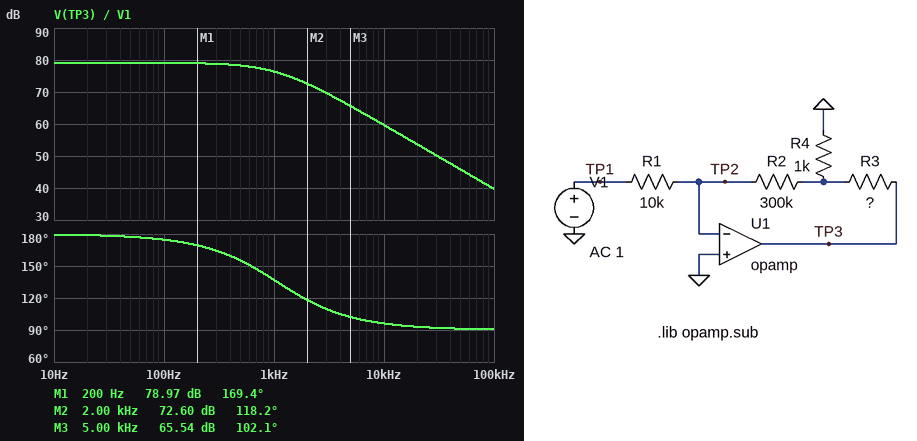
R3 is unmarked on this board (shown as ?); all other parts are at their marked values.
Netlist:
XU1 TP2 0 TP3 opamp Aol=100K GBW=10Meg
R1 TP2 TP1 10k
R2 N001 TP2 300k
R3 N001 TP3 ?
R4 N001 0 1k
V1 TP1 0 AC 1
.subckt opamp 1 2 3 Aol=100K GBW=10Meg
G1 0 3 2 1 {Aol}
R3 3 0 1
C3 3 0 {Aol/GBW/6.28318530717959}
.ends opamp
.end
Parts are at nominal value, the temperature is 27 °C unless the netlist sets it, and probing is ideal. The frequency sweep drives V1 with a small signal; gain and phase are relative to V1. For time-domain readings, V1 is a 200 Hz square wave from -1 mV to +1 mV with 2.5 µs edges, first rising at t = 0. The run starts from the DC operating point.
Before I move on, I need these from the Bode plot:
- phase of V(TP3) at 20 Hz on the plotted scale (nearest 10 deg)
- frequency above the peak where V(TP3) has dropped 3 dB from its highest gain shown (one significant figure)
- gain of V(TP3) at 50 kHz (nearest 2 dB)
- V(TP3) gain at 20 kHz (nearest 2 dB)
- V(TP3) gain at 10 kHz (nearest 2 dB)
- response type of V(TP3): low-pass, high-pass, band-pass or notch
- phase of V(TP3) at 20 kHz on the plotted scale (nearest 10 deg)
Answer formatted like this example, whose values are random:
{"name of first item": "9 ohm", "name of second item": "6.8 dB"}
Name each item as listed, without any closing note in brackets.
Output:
{"phase of V(TP3) at 20 Hz on the plotted scale": "180 deg", "frequency above the peak where V(TP3) has dropped 3 dB from its highest gain shown": "1 kHz", "gain of V(TP3) at 50 kHz": "46 dB", "V(TP3) gain at 20 kHz": "54 dB", "V(TP3) gain at 10 kHz": "60 dB", "response type of V(TP3): low-pass, high-pass, band-pass or notch": "low-pass", "phase of V(TP3) at 20 kHz on the plotted scale": "90 deg"}
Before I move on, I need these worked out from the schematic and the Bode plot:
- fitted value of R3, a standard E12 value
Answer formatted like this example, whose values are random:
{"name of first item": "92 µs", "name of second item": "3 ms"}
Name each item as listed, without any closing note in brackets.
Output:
{"fitted value of R3, a standard E12 value": "330 kΩ"}
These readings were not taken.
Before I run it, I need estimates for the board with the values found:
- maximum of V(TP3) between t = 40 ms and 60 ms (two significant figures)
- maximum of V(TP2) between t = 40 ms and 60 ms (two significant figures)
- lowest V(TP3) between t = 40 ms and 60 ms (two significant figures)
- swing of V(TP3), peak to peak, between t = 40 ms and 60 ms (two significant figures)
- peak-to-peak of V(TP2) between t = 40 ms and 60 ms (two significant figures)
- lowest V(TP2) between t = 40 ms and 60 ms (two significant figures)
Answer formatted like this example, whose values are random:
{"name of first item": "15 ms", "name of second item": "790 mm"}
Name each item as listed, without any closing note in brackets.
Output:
{"maximum of V(TP3) between t = 40 ms and 60 ms": "9.0 V", "maximum of V(TP2) between t = 40 ms and 60 ms": "1.8 mV", "lowest V(TP3) between t = 40 ms and 60 ms": "-9.0 V", "swing of V(TP3), peak to peak, between t = 40 ms and 60 ms": "18 V", "peak-to-peak of V(TP2) between t = 40 ms and 60 ms": "3.7 mV", "lowest V(TP2) between t = 40 ms and 60 ms": "-1.8 mV"}
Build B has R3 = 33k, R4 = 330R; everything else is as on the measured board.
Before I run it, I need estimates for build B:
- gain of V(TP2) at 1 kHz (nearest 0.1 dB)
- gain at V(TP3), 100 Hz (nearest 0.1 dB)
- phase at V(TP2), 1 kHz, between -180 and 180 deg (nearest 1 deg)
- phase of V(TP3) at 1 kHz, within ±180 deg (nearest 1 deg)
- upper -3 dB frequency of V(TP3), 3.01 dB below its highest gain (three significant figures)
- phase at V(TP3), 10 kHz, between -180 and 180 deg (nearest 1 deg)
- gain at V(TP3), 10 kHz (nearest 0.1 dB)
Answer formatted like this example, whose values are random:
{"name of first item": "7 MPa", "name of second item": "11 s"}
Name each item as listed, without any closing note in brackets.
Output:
{"gain of V(TP2) at 1 kHz": "-11.0 dB", "gain at V(TP3), 100 Hz": "69.4 dB", "phase at V(TP2), 1 kHz, between -180 and 180 deg": "67 deg", "phase of V(TP3) at 1 kHz, within ±180 deg": "163 deg", "upper -3 dB frequency of V(TP3), 3.01 dB below its highest gain": "3.29 kHz", "phase at V(TP3), 10 kHz, between -180 and 180 deg": "108 deg", "gain at V(TP3), 10 kHz": "59.3 dB"}
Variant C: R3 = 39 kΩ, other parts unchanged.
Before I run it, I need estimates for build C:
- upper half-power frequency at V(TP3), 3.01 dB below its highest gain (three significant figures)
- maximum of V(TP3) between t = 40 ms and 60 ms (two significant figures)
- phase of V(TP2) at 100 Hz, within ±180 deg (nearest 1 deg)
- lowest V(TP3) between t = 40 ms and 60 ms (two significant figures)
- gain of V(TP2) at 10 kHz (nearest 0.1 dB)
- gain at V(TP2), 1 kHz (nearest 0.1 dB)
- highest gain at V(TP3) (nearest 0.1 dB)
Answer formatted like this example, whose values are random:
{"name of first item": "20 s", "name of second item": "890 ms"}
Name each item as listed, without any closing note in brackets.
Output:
{"upper half-power frequency at V(TP3), 3.01 dB below its highest gain": "8.14 kHz", "maximum of V(TP3) between t = 40 ms and 60 ms": "1.2 V", "phase of V(TP2) at 100 Hz, within ±180 deg": "44 deg", "lowest V(TP3) between t = 40 ms and 60 ms": "-1.2 V", "gain of V(TP2) at 10 kHz": "-2.5 dB", "gain at V(TP2), 1 kHz": "-18.5 dB", "highest gain at V(TP3)": "61.5 dB"}
